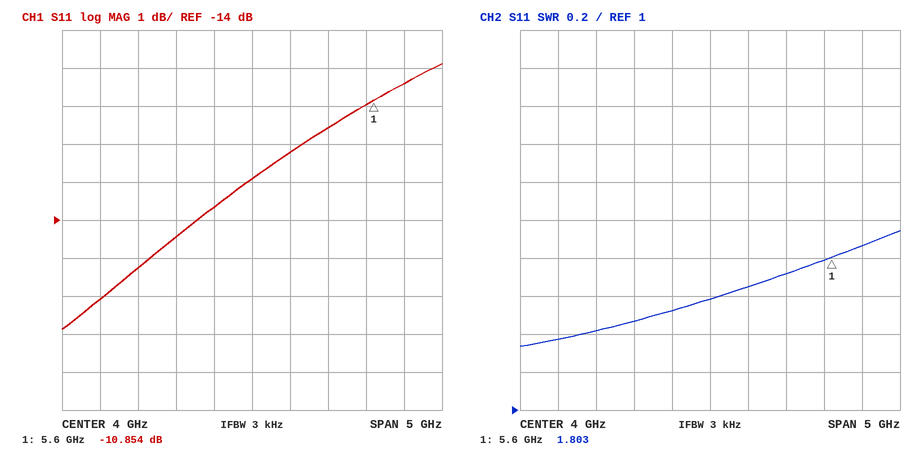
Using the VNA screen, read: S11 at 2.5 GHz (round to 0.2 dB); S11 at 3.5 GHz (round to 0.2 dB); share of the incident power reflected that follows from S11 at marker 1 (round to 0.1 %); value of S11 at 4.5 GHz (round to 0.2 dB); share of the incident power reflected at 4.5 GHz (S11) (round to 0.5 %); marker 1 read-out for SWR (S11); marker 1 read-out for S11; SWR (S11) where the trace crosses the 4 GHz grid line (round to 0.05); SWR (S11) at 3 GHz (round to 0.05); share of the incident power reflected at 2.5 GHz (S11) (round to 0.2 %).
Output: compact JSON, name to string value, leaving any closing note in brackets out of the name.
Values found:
{"S11 at 2.5 GHz": "-15.2 dB", "S11 at 3.5 GHz": "-13.6 dB", "share of the incident power reflected that follows from S11 at marker 1": "8.2 %", "value of S11 at 4.5 GHz": "-12.2 dB", "share of the incident power reflected at 4.5 GHz (S11)": "6.0 %", "marker 1 read-out for SWR": "1.803", "marker 1 read-out for S11": "-10.854 dB", "SWR (S11) where the trace crosses the 4 GHz grid line": "1.60", "SWR (S11) at 3 GHz": "1.45", "share of the incident power reflected at 2.5 GHz (S11)": "3.0 %"}
